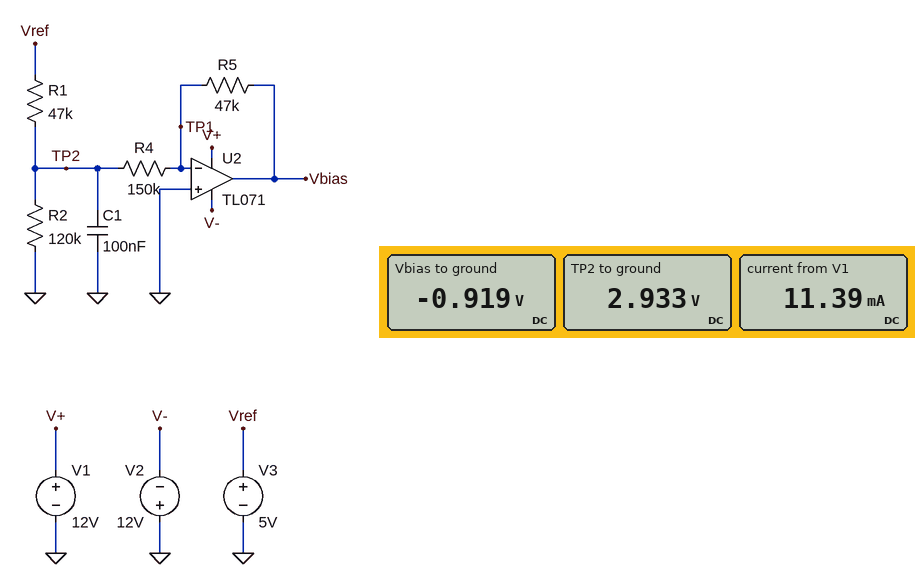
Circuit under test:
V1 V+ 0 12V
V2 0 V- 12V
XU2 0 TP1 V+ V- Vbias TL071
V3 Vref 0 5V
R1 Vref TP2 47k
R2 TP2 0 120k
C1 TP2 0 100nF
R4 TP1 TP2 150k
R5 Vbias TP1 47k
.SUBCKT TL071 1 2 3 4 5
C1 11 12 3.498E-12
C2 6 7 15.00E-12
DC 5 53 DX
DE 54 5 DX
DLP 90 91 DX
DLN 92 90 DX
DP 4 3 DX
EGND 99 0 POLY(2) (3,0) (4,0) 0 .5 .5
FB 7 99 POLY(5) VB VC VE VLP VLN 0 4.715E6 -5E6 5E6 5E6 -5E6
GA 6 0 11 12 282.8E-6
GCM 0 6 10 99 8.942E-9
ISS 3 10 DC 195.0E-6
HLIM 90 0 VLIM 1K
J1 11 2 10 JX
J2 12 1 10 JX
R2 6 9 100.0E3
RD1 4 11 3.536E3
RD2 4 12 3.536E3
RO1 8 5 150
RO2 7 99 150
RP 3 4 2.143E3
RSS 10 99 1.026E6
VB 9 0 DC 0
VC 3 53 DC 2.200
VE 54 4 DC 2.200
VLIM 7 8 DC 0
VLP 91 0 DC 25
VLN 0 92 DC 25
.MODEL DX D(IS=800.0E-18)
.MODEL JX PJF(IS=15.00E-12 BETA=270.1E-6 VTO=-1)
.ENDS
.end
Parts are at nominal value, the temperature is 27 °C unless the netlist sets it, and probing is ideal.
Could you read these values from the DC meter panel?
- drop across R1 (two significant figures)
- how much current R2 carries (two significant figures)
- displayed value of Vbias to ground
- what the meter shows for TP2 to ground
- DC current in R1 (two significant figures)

2.1 V
24 µA
-0.919 V
2.933 V
44 µA
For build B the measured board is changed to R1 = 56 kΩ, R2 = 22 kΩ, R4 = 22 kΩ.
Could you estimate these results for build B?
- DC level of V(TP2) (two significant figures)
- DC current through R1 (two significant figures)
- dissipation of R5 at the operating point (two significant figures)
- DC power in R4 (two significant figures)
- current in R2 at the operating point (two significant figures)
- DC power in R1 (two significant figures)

820 mV
75 µA
65 µW
31 µW
37 µA
310 µW
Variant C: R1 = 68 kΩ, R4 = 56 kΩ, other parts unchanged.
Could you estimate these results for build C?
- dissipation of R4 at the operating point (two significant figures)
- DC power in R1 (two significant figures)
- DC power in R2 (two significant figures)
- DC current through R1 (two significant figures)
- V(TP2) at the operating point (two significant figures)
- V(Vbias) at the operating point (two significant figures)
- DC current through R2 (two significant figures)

58 µW
150 µW
27 µW
47 µA
1.8 V
-1.5 V
15 µA
